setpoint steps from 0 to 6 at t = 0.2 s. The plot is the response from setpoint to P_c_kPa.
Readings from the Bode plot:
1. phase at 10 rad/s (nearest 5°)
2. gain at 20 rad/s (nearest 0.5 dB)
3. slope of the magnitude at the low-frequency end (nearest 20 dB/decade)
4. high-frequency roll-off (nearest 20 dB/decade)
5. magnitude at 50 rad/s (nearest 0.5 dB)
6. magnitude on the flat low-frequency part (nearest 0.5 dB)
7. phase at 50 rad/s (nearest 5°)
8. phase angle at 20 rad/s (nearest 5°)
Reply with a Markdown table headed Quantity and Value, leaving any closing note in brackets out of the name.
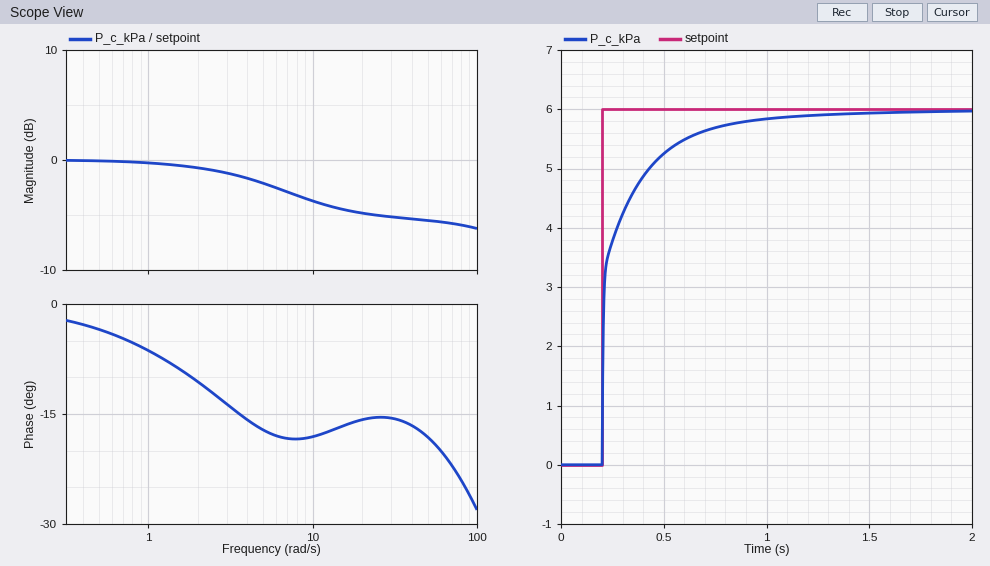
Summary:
| Quantity | Value |
|---|---|
| phase at 10 rad/s | -20° |
| gain at 20 rad/s | -5.0 dB |
| slope of the magnitude at the low-frequency end | 0 dB/decade |
| high-frequency roll-off | 0 dB/decade |
| magnitude at 50 rad/s | -5.5 dB |
| magnitude on the flat low-frequency part | 0.0 dB |
| phase at 50 rad/s | -20° |
| phase angle at 20 rad/s | -15° |
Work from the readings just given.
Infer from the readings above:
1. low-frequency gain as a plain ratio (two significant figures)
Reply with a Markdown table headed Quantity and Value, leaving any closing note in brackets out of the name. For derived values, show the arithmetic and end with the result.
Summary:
| Quantity | Value |
|---|---|
| low-frequency gain as a plain ratio | 10^(0 / 20) = 1.0 |
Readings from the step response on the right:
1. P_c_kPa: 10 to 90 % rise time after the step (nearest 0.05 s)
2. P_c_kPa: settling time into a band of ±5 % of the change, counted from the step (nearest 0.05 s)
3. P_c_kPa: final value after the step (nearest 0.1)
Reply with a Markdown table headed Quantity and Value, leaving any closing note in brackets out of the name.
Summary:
| Quantity | Value |
|---|---|
| P_c_kPa: 10 to 90 % rise time after the step | 0.35 s |
| P_c_kPa: settling time into a band of ±5 % of the change, counted from the step | 0.55 s |
| P_c_kPa: final value after the step | 6.0 |
